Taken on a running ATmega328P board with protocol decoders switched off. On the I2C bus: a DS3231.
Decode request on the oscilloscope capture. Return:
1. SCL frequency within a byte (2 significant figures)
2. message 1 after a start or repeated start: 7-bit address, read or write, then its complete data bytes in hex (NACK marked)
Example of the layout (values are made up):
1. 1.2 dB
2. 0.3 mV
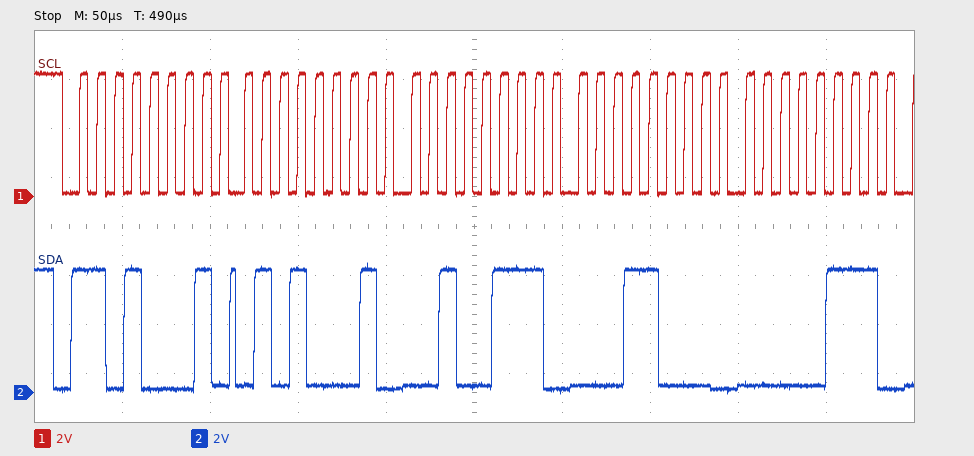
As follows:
1. 100 kHz
2. 0x68 read: 51 27 18 07
